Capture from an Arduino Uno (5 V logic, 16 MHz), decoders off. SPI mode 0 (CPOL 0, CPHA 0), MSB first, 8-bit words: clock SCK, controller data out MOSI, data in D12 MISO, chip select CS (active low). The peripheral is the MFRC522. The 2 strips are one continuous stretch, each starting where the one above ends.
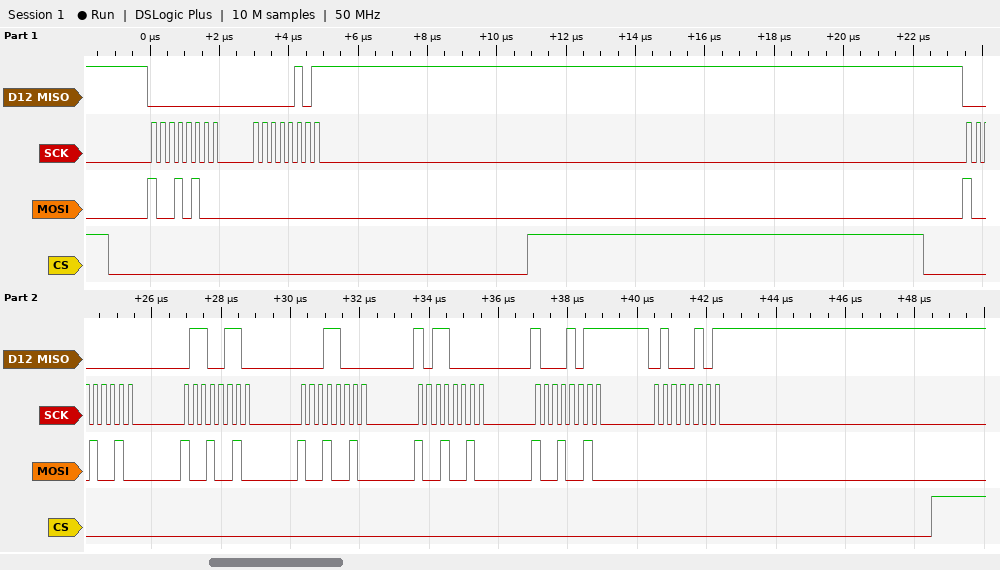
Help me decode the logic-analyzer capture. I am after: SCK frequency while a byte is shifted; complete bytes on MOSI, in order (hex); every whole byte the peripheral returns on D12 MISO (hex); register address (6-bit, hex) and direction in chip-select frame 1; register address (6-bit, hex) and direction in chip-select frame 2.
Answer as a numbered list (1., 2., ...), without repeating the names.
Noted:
1. 4 MHz
2. 94 00 92 92 92 92 92 00
3. 00 05 00 66 18 B0 8B 45
4. 0x0A read
5. 0x09 read
